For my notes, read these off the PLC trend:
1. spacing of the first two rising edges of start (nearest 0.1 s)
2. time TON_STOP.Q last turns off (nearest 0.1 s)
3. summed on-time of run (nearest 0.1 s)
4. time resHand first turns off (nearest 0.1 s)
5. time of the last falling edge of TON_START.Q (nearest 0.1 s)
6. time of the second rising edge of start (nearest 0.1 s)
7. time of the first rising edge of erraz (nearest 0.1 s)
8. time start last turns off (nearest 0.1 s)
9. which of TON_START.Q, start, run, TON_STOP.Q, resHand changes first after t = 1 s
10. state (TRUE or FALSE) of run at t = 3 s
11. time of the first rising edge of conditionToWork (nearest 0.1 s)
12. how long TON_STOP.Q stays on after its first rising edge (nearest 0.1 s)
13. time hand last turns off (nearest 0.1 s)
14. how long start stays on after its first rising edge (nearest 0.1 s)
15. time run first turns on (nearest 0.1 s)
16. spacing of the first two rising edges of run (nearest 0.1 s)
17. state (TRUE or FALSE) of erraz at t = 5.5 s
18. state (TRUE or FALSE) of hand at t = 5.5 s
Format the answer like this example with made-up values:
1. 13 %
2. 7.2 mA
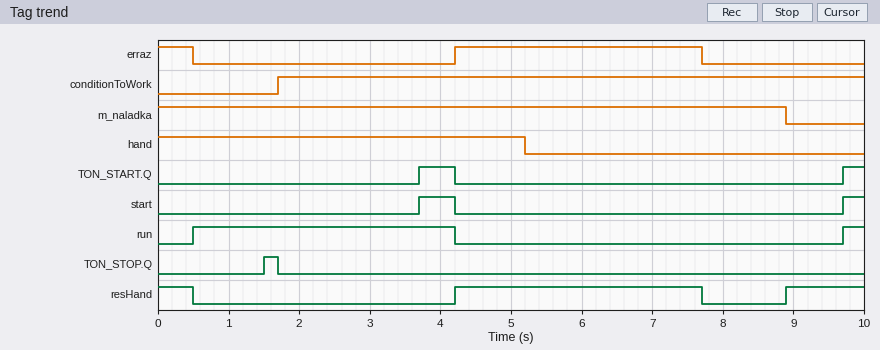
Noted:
1. 6.0 s
2. 1.7 s
3. 4.0 s
4. 0.5 s
5. 4.2 s
6. 9.7 s
7. 4.2 s
8. 4.2 s
9. TON_STOP.Q
10. TRUE
11. 1.7 s
12. 0.2 s
13. 5.2 s
14. 0.5 s
15. 0.5 s
16. 9.2 s
17. TRUE
18. FALSE
